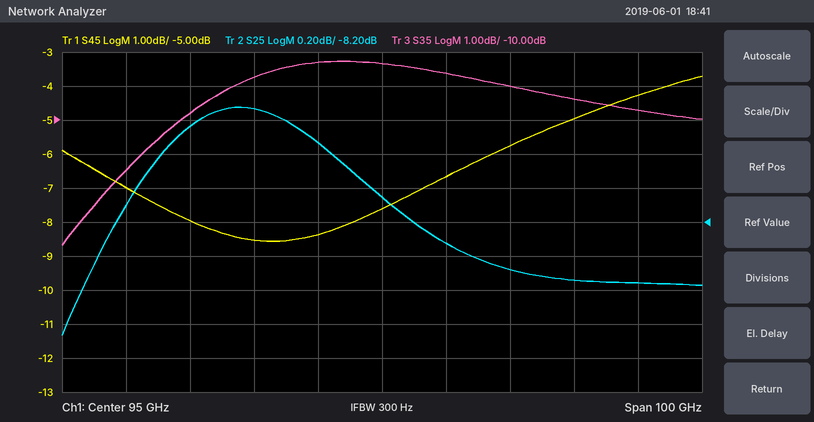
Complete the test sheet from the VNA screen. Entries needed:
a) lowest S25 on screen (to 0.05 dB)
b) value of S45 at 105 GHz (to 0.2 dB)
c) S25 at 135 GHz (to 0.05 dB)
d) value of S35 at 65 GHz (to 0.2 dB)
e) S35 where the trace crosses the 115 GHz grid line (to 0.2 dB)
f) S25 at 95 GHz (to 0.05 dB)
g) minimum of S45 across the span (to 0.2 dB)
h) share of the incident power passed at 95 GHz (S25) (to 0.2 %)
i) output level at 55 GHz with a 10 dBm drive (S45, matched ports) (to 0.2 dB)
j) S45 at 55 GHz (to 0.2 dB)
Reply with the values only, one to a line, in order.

-8.85 dB
-6.6 dB
-8.55 dB
-9.8 dB
-9.0 dB
-8.05 dB
-8.6 dB
15.6 %
3.0 dBm
-7.0 dB
